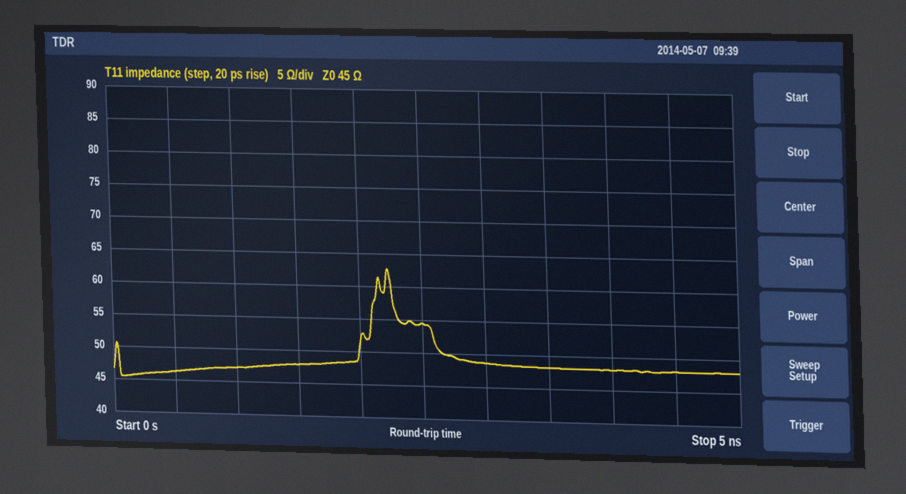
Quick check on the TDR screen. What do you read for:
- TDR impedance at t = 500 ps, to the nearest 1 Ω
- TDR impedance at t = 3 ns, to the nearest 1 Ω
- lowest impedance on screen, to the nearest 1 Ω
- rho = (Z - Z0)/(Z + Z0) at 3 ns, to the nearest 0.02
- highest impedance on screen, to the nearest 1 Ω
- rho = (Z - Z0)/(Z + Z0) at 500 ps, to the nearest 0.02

46 Ω
49 Ω
45 Ω
+0.04
63 Ω
+0.02
